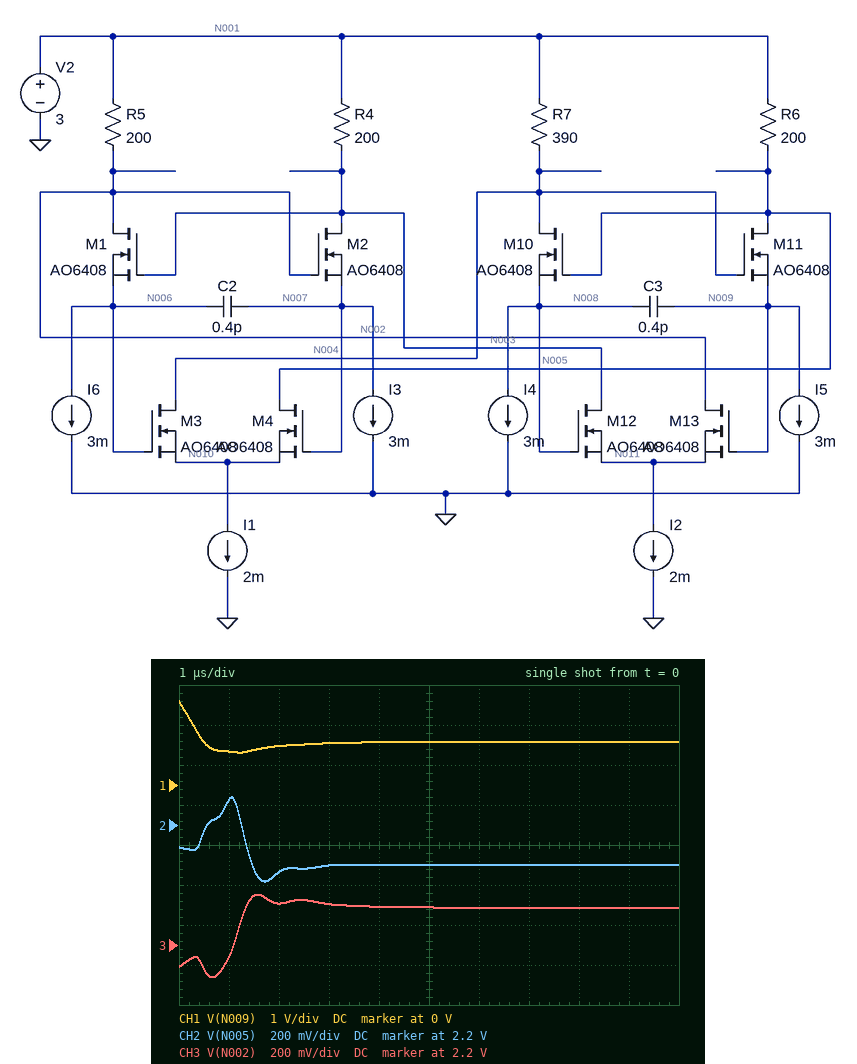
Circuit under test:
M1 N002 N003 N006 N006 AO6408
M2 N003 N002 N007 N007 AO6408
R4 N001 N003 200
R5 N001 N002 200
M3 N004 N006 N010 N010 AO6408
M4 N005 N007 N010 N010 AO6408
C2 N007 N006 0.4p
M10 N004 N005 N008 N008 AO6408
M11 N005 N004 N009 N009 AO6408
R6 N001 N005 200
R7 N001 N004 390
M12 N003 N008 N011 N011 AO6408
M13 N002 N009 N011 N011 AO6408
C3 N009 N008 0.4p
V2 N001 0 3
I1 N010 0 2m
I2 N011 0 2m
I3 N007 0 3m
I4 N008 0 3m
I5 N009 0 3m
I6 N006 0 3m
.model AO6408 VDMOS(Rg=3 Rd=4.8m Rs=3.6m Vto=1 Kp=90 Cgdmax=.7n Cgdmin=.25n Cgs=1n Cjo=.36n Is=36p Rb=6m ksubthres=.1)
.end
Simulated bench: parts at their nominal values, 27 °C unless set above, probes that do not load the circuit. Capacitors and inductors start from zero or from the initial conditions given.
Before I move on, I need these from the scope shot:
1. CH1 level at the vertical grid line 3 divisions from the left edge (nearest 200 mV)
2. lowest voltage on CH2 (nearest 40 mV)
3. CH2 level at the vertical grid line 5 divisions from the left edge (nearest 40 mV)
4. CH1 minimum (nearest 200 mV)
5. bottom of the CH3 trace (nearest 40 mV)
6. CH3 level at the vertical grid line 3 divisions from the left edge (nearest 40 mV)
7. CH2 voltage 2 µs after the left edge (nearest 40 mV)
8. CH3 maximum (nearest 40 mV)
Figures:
1.0 V
1.92 V
2.00 V
800 mV
2.04 V
2.40 V
1.96 V
2.44 V
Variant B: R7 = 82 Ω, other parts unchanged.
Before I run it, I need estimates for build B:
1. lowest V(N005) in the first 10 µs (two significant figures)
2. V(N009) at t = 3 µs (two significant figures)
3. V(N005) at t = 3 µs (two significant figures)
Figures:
2.1 V
1.8 V
2.4 V
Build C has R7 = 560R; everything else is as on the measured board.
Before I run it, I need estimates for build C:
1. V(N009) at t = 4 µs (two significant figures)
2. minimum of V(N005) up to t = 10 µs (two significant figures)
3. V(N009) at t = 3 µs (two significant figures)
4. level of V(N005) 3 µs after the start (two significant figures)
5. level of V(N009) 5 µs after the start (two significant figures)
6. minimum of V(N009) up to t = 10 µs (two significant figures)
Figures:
540 mV
2.0 V
500 mV
2.0 V
550 mV
440 mV
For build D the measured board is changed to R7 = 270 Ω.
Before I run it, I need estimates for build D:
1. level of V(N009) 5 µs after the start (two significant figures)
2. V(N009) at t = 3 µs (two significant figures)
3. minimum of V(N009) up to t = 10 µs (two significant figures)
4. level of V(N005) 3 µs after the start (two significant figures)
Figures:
1.2 V
1.3 V
1.1 V
1.9 V
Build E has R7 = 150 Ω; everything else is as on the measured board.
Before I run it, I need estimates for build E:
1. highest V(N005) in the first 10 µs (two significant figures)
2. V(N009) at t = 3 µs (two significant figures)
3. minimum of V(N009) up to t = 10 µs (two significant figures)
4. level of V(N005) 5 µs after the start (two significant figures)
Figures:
2.4 V
1.5 V
1.4 V
2.1 V
